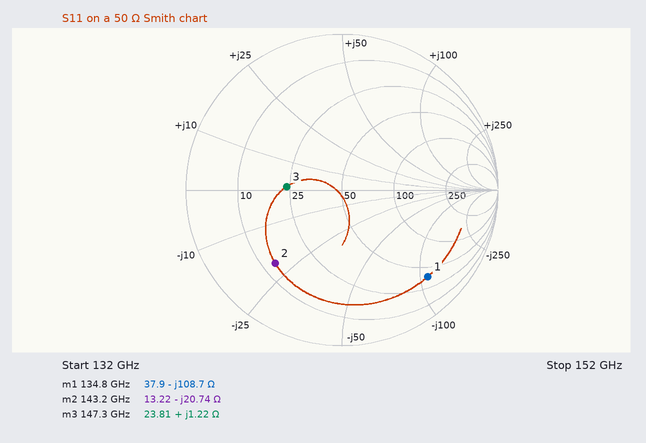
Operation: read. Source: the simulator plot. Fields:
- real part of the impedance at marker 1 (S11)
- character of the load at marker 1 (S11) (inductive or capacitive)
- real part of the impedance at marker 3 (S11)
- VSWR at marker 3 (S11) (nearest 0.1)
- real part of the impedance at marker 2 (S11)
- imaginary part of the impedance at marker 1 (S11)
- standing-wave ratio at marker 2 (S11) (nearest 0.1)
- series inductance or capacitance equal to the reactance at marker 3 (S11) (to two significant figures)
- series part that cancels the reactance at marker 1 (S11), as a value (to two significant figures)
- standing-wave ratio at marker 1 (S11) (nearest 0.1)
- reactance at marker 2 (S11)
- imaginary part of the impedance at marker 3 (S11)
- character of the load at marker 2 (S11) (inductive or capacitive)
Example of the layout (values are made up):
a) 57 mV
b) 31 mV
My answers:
a) 37.9 Ω
b) capacitive
c) 23.81 Ω
d) 2.1
e) 13.22 Ω
f) -108.7 Ω
g) 4.5
h) 1.3 pH
i) 130 pH
j) 8.2
k) -20.74 Ω
l) +1.22 Ω
m) capacitive
